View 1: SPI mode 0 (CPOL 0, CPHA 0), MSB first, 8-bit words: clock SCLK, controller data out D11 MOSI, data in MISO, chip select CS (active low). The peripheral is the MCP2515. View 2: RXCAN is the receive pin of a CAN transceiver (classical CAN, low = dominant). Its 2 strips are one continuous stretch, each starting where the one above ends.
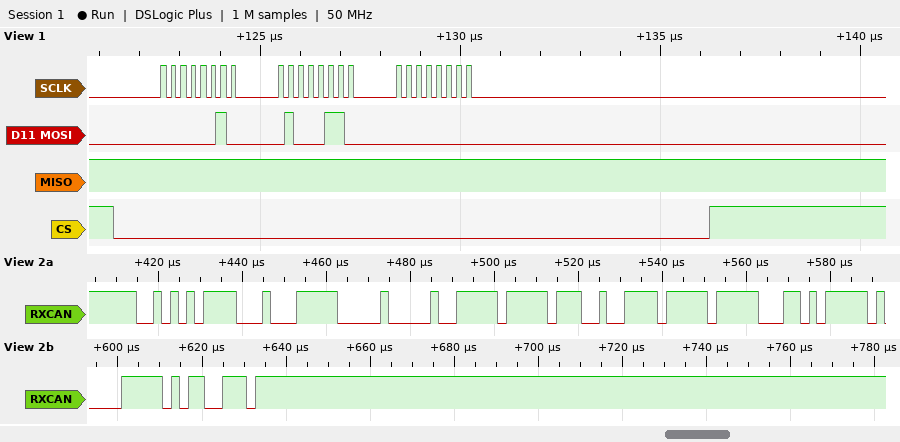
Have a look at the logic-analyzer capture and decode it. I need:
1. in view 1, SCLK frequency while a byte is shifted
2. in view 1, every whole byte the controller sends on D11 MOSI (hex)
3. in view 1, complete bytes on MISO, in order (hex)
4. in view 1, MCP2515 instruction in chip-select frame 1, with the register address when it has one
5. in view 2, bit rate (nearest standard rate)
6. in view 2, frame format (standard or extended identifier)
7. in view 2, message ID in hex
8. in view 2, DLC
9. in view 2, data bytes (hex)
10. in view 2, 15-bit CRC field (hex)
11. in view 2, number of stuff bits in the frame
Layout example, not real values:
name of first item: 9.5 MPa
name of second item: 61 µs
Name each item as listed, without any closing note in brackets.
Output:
in view 1, SCLK frequency while a byte is shifted: 4 MHz
in view 1, every whole byte the controller sends on D11 MOSI: 02 46 00
in view 1, complete bytes on MISO, in order: FF FF FF
in view 1, MCP2515 instruction in chip-select frame 1, with the register address when it has one: WRITE 0x46
in view 2, bit rate: 500 kbit/s
in view 2, frame format: standard
in view 2, message ID in hex: 0x2AF
in view 2, DLC: 8
in view 2, data bytes: F8 00 FF F9 3D FF 9A FC
in view 2, 15-bit CRC field: 0x1FB3
in view 2, number of stuff bits in the frame: 9
